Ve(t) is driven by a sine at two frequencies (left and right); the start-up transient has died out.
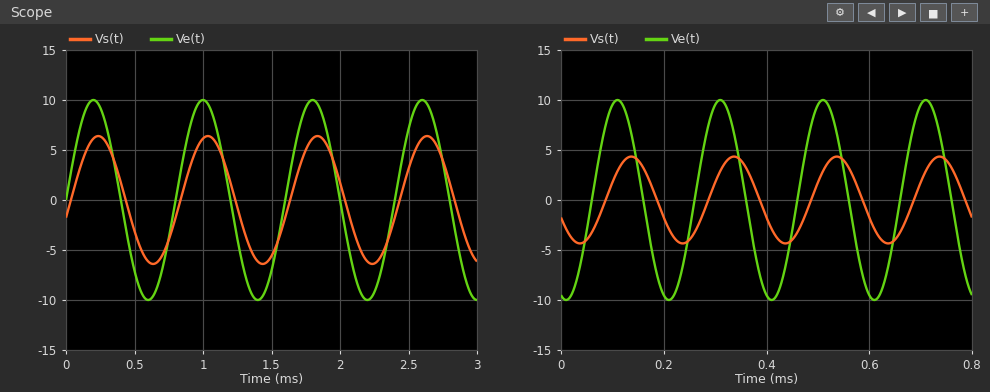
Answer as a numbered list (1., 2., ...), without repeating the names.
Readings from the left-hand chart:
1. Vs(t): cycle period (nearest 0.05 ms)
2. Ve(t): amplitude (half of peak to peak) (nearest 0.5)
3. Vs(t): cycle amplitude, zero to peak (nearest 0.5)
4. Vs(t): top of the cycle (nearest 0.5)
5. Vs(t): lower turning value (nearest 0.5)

1. 0.80 ms
2. 10.0
3. 6.5
4. 6.5
5. -6.5
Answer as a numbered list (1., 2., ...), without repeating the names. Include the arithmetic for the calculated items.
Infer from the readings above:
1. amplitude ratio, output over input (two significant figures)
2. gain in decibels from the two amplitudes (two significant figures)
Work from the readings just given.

1. 6.5 / 10 = 0.65
2. 20 log10(6.5 / 10) = -3.7 dB
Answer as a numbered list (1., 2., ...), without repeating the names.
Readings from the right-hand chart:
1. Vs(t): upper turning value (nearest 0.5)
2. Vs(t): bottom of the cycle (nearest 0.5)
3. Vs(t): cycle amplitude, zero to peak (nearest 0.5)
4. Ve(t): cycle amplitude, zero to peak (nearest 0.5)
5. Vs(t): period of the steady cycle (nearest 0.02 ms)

1. 4.5
2. -4.5
3. 4.5
4. 10.0
5. 0.20 ms
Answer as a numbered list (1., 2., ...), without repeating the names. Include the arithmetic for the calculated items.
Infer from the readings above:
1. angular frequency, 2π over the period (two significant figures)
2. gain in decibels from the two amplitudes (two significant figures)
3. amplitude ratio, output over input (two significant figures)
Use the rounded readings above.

1. 2π / 0.2 = 31 rad/ms
2. 20 log10(4.5 / 10) = -6.9 dB
3. 4.5 / 10 = 0.45
